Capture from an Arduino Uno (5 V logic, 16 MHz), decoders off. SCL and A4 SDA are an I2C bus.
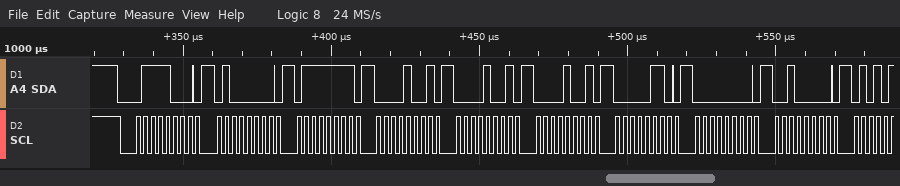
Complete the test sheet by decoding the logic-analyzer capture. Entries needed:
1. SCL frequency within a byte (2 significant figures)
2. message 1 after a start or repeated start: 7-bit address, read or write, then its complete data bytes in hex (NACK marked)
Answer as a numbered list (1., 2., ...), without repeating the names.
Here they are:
1. 400 kHz
2. 0x3C write: 40 7F 09 09 09 06 00 20
